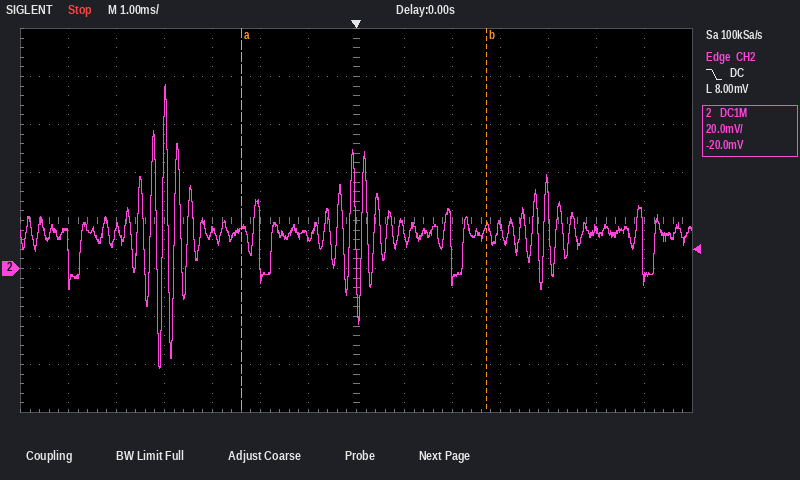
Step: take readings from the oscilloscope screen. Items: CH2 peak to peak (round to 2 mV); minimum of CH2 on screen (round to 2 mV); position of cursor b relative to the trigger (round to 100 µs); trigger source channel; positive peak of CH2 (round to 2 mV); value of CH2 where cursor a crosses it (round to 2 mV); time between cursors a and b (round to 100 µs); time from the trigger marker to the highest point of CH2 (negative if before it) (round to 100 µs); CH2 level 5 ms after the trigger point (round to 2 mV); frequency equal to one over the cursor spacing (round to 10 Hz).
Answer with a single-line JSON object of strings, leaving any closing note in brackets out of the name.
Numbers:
{"CH2 peak to peak": "118 mV", "minimum of CH2 on screen": "-42 mV", "position of cursor b relative to the trigger": "+2.7 ms", "trigger source channel": "CH2", "positive peak of CH2": "76 mV", "value of CH2 where cursor a crosses it": "16 mV", "time between cursors a and b": "5.1 ms", "time from the trigger marker to the highest point of CH2 (negative if before it)": "-4.0 ms", "CH2 level 5 ms after the trigger point": "16 mV", "frequency equal to one over the cursor spacing": "200 Hz"}
